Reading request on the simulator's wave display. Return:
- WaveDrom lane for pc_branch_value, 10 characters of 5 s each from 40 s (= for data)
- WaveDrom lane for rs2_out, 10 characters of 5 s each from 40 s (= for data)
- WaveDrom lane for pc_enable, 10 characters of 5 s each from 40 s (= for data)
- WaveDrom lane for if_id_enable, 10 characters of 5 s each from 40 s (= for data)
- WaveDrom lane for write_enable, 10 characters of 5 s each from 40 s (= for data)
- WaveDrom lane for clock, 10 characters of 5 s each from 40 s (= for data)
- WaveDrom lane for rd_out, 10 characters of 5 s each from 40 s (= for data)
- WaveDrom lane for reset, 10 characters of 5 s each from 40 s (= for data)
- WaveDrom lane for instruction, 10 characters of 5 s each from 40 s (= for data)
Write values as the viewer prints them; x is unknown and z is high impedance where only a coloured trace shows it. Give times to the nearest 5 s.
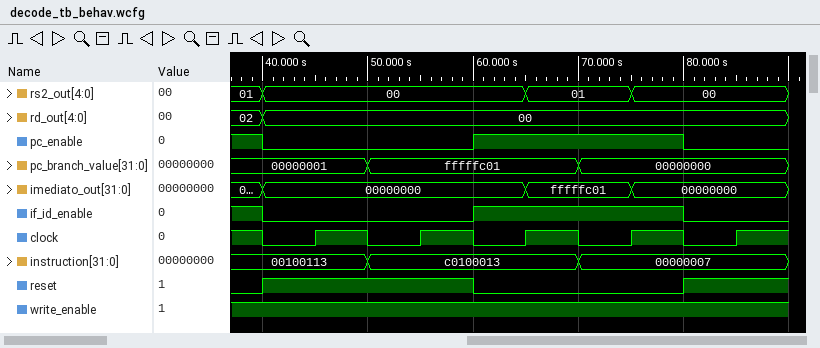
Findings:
{name: 'pc_branch_value', wave: '=.=...=...', data: '00000001 fffffc01 00000000'}
{name: 'rs2_out', wave: '=....=.=..', data: '00 01 00'}
{name: 'pc_enable', wave: '0...1...0.'}
{name: 'if_id_enable', wave: '0...1...0.'}
{name: 'write_enable', wave: '1.........'}
{name: 'clock', wave: '0101010101'}
{name: 'rd_out', wave: '=.........', data: '00'}
{name: 'reset', wave: '1...0...1.'}
{name: 'instruction', wave: '=.=...=...', data: '00100113 c0100013 00000007'}
